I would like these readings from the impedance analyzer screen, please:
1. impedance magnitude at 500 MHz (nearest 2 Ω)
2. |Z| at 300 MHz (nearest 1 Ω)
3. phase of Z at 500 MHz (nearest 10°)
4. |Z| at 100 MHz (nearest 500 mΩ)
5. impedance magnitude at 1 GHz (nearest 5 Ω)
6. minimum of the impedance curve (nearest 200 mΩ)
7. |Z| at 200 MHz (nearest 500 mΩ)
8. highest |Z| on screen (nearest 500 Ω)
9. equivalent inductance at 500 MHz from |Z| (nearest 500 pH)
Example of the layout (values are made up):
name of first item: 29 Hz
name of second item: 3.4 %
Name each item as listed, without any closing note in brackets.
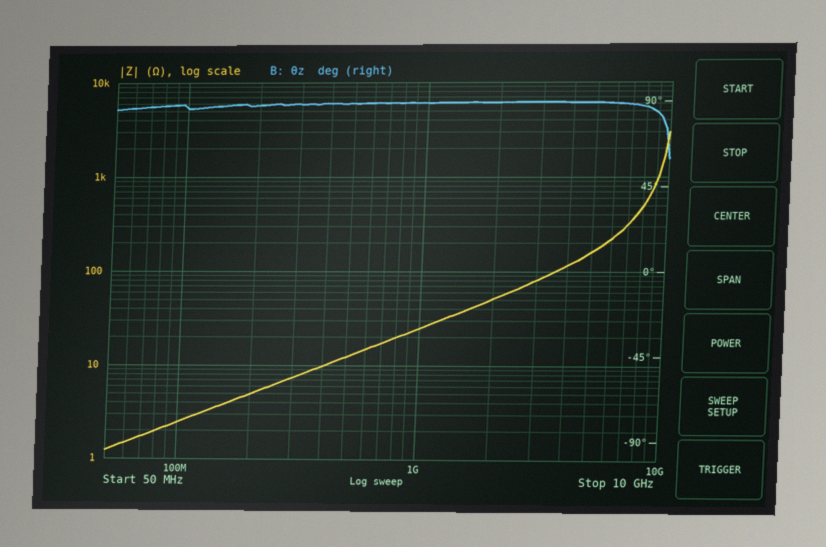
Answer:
impedance magnitude at 500 MHz: 12 Ω
|Z| at 300 MHz: 7 Ω
phase of Z at 500 MHz: 90°
|Z| at 100 MHz: 2.5 Ω
impedance magnitude at 1 GHz: 25 Ω
minimum of the impedance curve: 1.2 Ω
|Z| at 200 MHz: 5.0 Ω
highest |Z| on screen: 3.0 kΩ
equivalent inductance at 500 MHz from |Z|: 4.0 nH
